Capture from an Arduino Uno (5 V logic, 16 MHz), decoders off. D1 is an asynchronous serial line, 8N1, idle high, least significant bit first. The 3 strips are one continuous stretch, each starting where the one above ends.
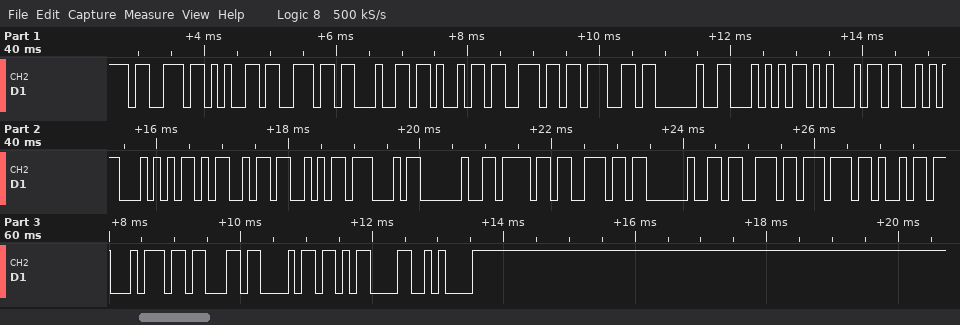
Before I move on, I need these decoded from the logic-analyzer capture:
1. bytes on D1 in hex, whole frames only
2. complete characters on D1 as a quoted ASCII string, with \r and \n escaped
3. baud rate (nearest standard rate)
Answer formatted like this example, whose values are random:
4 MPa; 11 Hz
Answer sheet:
73 65 6E 64 69 6E 67 20 54 45 53 54 4D 53 47 20 6F 6E 20 73 77 69 74 63 68 0D 0A; "sending TESTMSG on switch\r\n"; 9600 baud
